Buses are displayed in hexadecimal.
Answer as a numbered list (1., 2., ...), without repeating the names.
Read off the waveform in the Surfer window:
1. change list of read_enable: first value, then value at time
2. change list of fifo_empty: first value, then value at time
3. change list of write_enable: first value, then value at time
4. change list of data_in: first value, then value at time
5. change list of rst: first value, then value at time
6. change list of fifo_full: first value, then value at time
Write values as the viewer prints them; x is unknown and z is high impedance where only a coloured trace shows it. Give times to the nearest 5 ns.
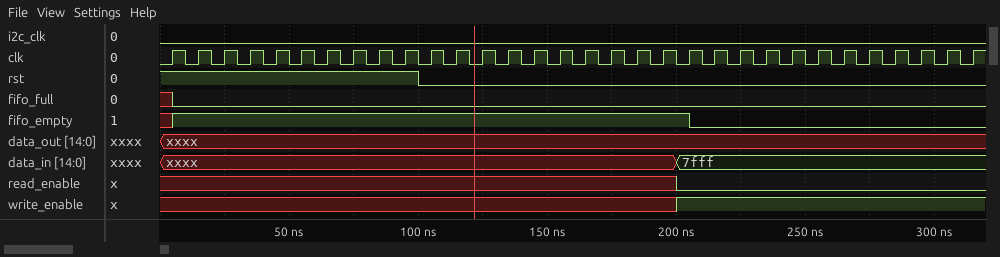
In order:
1. x, 0 at 200 ns
2. x, 1 at 5 ns, 0 at 205 ns
3. x, 1 at 200 ns
4. xxxx, 7fff at 200 ns
5. 1, 0 at 100 ns
6. x, 0 at 5 ns
